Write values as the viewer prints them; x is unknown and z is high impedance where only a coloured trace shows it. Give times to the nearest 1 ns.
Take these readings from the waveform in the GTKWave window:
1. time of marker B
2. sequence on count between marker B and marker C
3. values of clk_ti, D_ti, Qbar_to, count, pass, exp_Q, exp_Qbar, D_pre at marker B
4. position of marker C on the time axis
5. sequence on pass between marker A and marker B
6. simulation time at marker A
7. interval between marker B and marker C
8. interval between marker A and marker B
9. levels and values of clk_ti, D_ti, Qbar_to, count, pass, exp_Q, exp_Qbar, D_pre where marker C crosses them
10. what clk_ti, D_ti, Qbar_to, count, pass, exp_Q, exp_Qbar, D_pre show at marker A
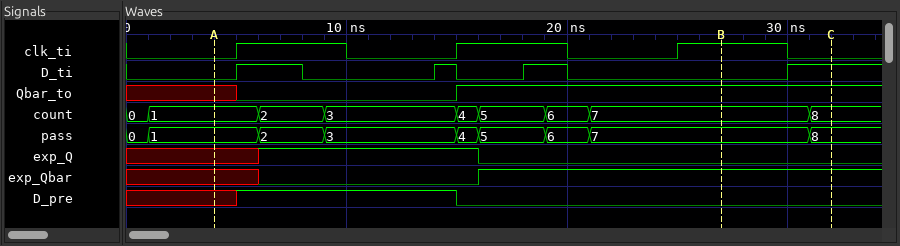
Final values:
27 ns
7, 8
clk_ti=1, D_ti=0, Qbar_to=1, count=7, pass=7, exp_Q=0, exp_Qbar=1, D_pre=0
32 ns
1, 2, 3, 4, 5, 6, 7
4 ns
5 ns
23 ns
clk_ti=0, D_ti=1, Qbar_to=1, count=8, pass=8, exp_Q=0, exp_Qbar=1, D_pre=0
clk_ti=0, D_ti=0, Qbar_to=x, count=1, pass=1, exp_Q=x, exp_Qbar=x, D_pre=x
